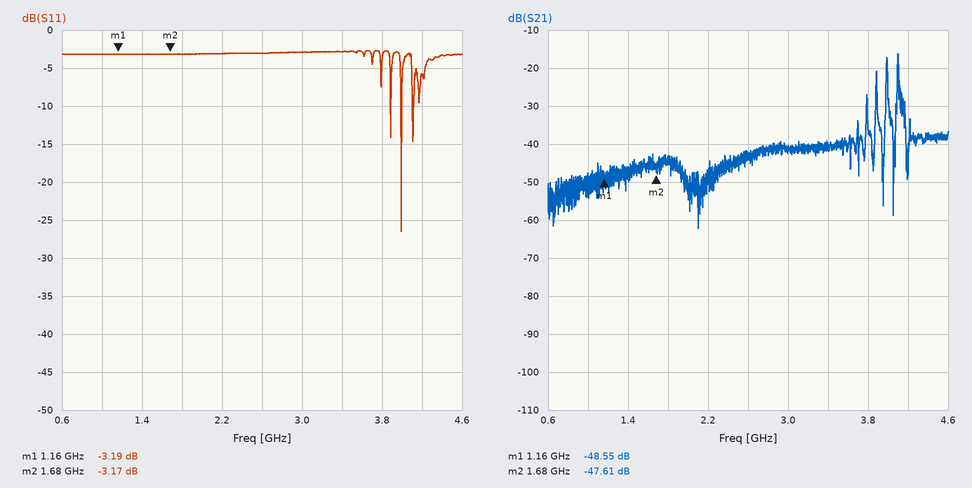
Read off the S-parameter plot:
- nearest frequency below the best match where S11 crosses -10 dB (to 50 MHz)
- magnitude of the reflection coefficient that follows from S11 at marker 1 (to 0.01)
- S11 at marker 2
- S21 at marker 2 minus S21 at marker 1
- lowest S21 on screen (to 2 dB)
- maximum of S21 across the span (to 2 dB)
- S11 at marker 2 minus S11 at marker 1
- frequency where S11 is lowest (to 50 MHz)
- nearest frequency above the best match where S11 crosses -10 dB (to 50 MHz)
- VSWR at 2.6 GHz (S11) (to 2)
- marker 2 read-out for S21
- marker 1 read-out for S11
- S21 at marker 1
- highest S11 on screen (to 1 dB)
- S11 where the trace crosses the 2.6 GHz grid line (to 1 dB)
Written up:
4.00 GHz
0.69
-3.17 dB
0.94 dB
-62 dB
-16 dB
0.02 dB
4.00 GHz
4.00 GHz
6
-47.61 dB
-3.19 dB
-48.55 dB
-3 dB
-3 dB
